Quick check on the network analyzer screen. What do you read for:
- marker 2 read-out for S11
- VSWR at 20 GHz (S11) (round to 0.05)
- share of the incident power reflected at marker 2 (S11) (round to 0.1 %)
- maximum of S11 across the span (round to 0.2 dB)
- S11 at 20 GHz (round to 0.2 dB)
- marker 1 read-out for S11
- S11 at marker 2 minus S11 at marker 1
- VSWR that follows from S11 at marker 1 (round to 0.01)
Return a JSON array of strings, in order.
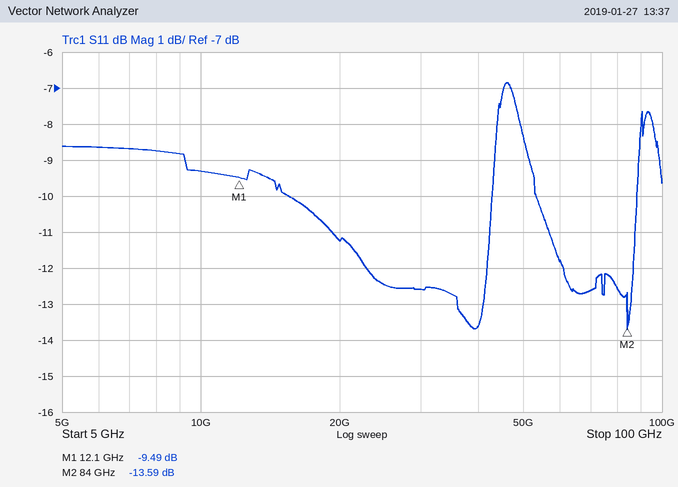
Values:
["-13.59 dB", "1.75", "4.4 %", "-6.8 dB", "-11.2 dB", "-9.49 dB", "-4.10 dB", "2.01"]
